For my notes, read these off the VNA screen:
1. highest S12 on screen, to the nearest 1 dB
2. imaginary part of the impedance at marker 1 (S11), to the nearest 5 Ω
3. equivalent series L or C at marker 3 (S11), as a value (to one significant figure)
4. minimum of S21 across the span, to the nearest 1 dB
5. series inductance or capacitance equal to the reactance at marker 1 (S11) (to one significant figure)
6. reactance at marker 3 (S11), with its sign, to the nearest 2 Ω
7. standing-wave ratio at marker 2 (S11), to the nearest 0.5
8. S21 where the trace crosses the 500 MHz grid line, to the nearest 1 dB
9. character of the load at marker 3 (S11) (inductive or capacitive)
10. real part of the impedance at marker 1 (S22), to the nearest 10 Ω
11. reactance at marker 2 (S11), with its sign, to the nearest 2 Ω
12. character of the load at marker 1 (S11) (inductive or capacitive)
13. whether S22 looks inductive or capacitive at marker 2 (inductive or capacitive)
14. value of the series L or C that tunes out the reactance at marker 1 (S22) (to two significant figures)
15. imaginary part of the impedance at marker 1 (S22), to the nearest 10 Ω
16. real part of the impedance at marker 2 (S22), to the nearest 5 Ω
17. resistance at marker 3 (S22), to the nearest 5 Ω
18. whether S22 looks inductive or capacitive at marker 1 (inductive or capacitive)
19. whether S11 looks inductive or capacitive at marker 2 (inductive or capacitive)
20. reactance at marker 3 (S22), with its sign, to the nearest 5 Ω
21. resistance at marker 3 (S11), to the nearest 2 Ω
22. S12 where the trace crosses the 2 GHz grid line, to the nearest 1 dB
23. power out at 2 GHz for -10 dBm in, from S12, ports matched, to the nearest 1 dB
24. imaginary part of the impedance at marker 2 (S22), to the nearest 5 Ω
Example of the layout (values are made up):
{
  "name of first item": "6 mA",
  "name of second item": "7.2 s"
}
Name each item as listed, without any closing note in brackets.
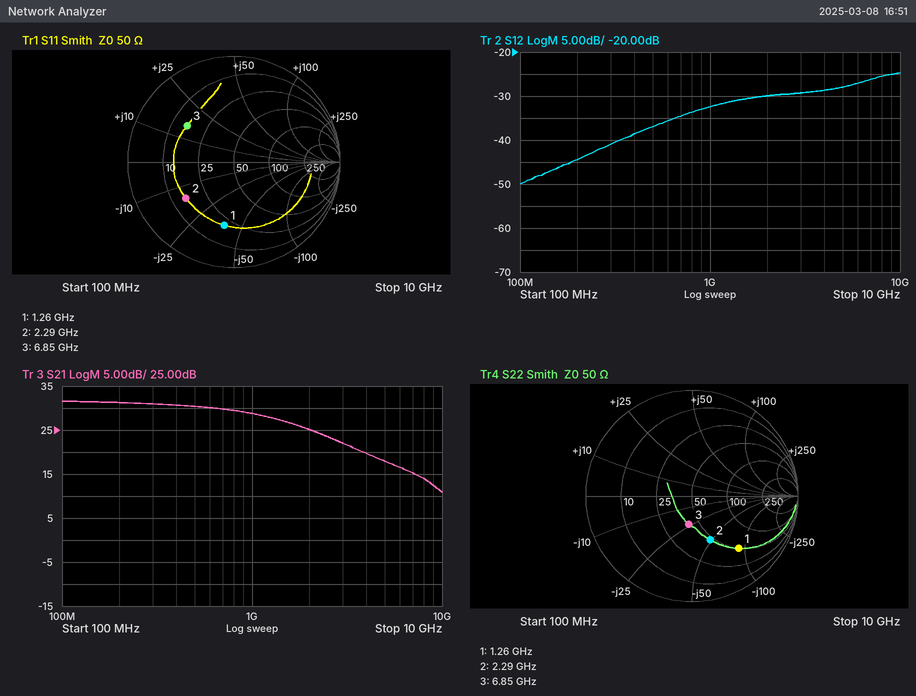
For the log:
{
  "highest S12 on screen, to the nearest 1 dB": "-25 dB",
  "imaginary part of the impedance at marker 1 (S11), to the nearest 5 Ω": "-40 Ω",
  "equivalent series L or C at marker 3 (S11), as a value": "400 pH",
  "minimum of S21 across the span, to the nearest 1 dB": "11 dB",
  "series inductance or capacitance equal to the reactance at marker 1 (S11)": "3 pF",
  "reactance at marker 3 (S11), with its sign, to the nearest 2 Ω": "+16 Ω",
  "standing-wave ratio at marker 2 (S11), to the nearest 0.5": "3.5",
  "S21 where the trace crosses the 500 MHz grid line, to the nearest 1 dB": "30 dB",
  "character of the load at marker 3 (S11)": "inductive",
  "real part of the impedance at marker 1 (S22), to the nearest 10 Ω": "50 Ω",
  "reactance at marker 2 (S11), with its sign, to the nearest 2 Ω": "-16 Ω",
  "character of the load at marker 1 (S11)": "capacitive",
  "whether S22 looks inductive or capacitive at marker 2": "capacitive",
  "value of the series L or C that tunes out the reactance at marker 1 (S22)": "11 nH",
  "imaginary part of the impedance at marker 1 (S22), to the nearest 10 Ω": "-90 Ω",
  "real part of the impedance at marker 2 (S22), to the nearest 5 Ω": "45 Ω",
  "resistance at marker 3 (S22), to the nearest 5 Ω": "40 Ω",
  "whether S22 looks inductive or capacitive at marker 1": "capacitive",
  "whether S11 looks inductive or capacitive at marker 2": "capacitive",
  "reactance at marker 3 (S22), with its sign, to the nearest 5 Ω": "-25 Ω",
  "resistance at marker 3 (S11), to the nearest 2 Ω": "16 Ω",
  "S12 where the trace crosses the 2 GHz grid line, to the nearest 1 dB": "-30 dB",
  "power out at 2 GHz for -10 dBm in, from S12, ports matched, to the nearest 1 dB": "-40 dBm",
  "imaginary part of the impedance at marker 2 (S22), to the nearest 5 Ω": "-50 Ω"
}
